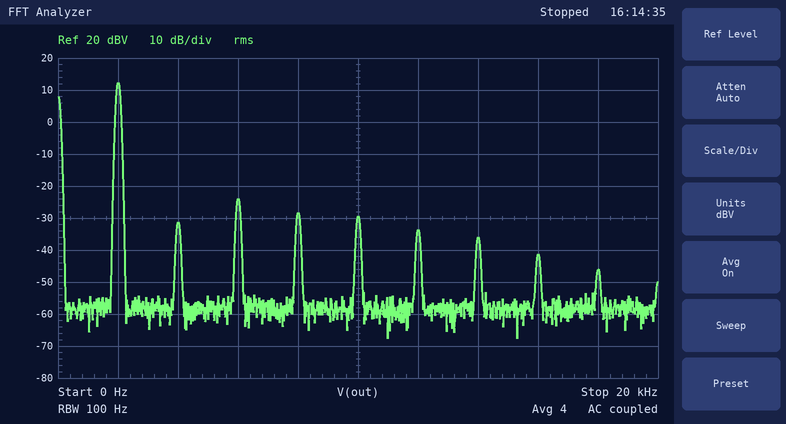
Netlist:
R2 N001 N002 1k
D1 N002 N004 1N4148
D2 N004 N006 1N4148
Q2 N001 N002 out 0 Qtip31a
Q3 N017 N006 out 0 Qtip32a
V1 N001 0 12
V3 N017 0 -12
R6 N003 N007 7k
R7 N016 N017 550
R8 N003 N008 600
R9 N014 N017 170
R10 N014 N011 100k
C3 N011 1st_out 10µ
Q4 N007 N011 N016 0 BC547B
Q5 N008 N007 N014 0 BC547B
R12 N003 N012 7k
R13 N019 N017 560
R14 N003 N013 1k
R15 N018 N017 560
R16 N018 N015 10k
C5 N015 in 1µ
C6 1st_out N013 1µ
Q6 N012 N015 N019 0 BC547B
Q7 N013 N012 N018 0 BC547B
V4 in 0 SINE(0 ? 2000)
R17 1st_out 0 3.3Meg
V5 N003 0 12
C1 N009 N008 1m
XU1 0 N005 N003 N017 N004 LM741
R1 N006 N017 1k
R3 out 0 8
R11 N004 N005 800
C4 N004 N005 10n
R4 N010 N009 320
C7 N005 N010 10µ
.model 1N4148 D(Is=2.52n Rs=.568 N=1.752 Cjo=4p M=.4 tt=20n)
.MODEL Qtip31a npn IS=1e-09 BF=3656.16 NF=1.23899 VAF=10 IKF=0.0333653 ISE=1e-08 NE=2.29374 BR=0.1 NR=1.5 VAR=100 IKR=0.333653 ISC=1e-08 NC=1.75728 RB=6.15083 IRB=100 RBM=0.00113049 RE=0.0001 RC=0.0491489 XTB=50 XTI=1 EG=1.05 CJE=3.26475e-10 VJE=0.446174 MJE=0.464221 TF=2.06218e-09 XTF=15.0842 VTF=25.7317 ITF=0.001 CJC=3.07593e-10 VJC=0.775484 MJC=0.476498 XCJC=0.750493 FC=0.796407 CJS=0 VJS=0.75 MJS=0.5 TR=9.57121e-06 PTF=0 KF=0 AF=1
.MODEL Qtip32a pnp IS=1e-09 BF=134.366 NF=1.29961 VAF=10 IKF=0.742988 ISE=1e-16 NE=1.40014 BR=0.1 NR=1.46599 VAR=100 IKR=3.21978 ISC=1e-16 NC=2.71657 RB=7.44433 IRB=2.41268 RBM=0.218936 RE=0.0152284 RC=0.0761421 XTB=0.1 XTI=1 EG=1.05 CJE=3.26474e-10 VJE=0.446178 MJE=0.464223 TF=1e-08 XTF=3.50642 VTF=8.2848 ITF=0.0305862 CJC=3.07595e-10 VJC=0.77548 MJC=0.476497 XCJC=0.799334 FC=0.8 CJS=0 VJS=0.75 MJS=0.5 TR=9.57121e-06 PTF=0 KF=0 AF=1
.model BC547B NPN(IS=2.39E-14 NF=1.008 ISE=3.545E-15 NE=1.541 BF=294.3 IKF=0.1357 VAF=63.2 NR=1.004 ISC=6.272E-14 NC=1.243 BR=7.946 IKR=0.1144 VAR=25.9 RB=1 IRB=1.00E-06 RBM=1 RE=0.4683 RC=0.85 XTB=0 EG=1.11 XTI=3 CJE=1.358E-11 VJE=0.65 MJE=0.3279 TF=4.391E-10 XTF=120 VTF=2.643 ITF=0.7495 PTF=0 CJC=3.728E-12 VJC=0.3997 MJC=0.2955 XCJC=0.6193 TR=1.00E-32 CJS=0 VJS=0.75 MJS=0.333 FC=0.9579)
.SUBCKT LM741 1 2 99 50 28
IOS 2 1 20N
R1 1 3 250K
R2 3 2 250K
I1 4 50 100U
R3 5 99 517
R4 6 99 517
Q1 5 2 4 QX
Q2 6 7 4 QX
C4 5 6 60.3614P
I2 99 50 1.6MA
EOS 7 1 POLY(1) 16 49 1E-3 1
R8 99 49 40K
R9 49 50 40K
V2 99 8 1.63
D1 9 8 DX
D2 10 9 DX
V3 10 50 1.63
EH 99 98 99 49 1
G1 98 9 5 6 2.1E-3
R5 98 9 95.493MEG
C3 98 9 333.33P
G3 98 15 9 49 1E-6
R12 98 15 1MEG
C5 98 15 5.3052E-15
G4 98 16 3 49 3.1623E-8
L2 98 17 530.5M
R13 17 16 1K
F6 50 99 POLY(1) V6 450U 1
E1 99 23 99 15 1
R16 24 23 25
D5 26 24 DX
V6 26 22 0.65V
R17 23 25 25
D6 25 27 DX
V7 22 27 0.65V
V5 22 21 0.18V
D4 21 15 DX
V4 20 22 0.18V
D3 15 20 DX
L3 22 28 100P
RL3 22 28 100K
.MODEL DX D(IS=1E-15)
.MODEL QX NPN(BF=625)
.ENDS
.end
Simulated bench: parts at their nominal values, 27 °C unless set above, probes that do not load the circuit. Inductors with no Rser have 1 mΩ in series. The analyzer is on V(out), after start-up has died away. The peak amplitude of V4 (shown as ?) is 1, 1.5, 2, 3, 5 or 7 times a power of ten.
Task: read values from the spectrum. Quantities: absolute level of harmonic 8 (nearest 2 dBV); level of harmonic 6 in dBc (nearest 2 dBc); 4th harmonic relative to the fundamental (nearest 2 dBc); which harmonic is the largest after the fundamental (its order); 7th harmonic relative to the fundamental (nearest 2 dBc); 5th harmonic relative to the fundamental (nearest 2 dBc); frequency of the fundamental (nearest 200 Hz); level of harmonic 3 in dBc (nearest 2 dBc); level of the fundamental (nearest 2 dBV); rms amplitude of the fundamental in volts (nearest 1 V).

-42 dBV
-46 dBc
-40 dBc
3
-48 dBc
-42 dBc
2.0 kHz
-36 dBc
12 dBV
4 V
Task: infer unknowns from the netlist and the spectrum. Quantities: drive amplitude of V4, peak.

10 mV
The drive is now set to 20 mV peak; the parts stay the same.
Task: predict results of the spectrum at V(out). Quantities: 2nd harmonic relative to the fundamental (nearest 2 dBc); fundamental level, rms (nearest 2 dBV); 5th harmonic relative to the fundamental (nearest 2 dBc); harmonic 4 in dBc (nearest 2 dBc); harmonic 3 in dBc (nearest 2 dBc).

-46 dBc
14 dBV
-24 dBc
-44 dBc
-12 dBc
